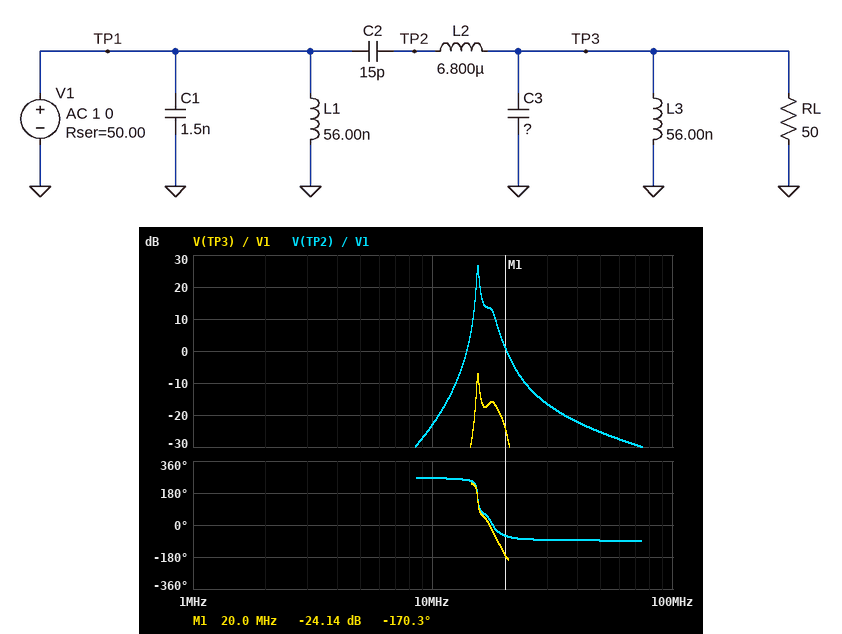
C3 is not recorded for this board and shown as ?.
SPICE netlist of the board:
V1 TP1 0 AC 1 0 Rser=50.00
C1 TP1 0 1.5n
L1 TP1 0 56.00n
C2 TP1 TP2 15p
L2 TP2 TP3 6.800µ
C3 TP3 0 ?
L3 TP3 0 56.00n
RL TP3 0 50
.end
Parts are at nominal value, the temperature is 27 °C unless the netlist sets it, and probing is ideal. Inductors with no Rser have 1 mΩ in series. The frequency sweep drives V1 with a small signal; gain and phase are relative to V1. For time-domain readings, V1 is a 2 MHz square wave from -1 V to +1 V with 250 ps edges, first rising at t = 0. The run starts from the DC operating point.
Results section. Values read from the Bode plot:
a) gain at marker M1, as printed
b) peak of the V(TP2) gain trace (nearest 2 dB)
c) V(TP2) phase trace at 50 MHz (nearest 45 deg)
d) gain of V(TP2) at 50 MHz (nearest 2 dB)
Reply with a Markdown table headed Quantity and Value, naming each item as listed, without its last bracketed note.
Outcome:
| Quantity | Value |
|---|---|
| gain at marker M1, as printed | -24.14 dB |
| peak of the V(TP2) gain trace | 26 dB |
| V(TP2) phase trace at 50 MHz | -90 deg |
| gain of V(TP2) at 50 MHz | -26 dB |
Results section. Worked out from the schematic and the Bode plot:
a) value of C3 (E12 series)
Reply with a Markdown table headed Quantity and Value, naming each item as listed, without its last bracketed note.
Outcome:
| Quantity | Value |
|---|---|
| value of C3 | 1.2 nF |
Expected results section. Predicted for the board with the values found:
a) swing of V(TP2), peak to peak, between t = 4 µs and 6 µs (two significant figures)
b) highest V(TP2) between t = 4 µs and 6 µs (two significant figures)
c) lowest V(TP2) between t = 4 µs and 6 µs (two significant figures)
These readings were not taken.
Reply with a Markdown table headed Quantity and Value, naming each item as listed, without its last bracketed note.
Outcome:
| Quantity | Value |
|---|---|
| swing of V(TP2), peak to peak, between t = 4 µs and 6 µs | 1.3 V |
| highest V(TP2) between t = 4 µs and 6 µs | 660 mV |
| lowest V(TP2) between t = 4 µs and 6 µs | -660 mV |
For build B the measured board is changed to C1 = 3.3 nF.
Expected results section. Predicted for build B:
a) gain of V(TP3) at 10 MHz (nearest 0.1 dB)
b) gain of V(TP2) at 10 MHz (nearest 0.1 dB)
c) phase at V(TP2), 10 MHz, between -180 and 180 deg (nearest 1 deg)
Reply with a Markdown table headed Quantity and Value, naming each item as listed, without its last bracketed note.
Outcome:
| Quantity | Value |
|---|---|
| gain of V(TP3) at 10 MHz | -54.2 dB |
| gain of V(TP2) at 10 MHz | -15.1 dB |
| phase at V(TP2), 10 MHz, between -180 and 180 deg | -105 deg |
